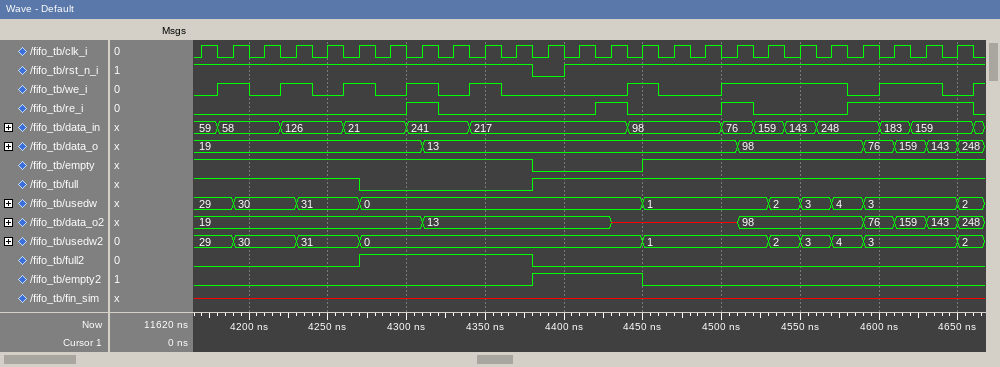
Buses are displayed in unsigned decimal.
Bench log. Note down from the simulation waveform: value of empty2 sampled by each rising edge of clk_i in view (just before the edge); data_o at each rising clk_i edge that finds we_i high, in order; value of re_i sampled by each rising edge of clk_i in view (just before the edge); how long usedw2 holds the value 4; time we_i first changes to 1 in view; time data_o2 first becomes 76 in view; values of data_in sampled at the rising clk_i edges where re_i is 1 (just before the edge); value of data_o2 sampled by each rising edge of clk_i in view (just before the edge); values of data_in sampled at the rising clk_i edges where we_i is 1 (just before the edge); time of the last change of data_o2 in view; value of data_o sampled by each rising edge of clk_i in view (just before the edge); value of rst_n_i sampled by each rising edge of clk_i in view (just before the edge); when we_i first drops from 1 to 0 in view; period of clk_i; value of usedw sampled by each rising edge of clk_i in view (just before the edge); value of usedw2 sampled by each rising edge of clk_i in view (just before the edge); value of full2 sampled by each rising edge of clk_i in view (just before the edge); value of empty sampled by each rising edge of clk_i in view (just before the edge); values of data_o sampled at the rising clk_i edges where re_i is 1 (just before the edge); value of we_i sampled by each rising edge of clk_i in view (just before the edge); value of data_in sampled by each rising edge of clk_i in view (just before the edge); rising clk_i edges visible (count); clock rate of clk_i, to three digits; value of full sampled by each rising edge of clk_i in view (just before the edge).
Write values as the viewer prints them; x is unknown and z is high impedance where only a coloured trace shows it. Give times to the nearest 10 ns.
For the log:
0 0 0 0 0 0 0 0 0 0 0 1 1 1 1 0 0 0 0 0 0 0 0 0 0
19, 19, 19, 19, 13, 13, 13, 98, 98, 98, 76, 159
0 0 0 0 0 0 0 1 0 0 0 0 0 1 0 0 0 1 0 0 0 1 1 1 1
20 ns
4180 ns
4590 ns
241, 217, 76, 248, 183, 159, 159
19, 19, 19, 19, 19, 19, 19, 19, 13, 13, 13, 13, 13, 13, x, x, x, x, 98, 98, 98, 98, 76, 159, 143
58, 126, 21, 241, 217, 98, 76, 159, 143, 248, 183, 159
4650 ns
19, 19, 19, 19, 19, 19, 19, 19, 13, 13, 13, 13, 13, 13, 13, 13, 13, 13, 98, 98, 98, 98, 76, 159, 143
1 1 1 1 1 1 1 1 1 1 1 0 1 1 1 1 1 1 1 1 1 1 1 1 1
4200 ns
20 ns
29, 29, 30, 30, 31, 31, 0, 0, 0, 0, 0, 0, 0, 0, 0, 1, 1, 1, 1, 2, 3, 4, 3, 3, 3
29, 29, 30, 30, 31, 31, 0, 0, 0, 0, 0, 0, 0, 0, 0, 1, 1, 1, 1, 2, 3, 4, 3, 3, 3
0 0 0 0 0 0 1 1 1 1 1 0 0 0 0 0 0 0 0 0 0 0 0 0 0
1 1 1 1 1 1 1 1 1 1 1 0 0 0 0 1 1 1 1 1 1 1 1 1 1
19, 13, 13, 98, 76, 159, 143
0 1 0 1 0 1 0 1 0 1 0 0 0 0 1 0 0 1 1 1 1 0 1 1 0
59, 58, 58, 126, 126, 21, 21, 241, 241, 217, 217, 217, 217, 217, 98, 98, 98, 76, 159, 143, 248, 248, 183, 159, 159
25
50.0 MHz
1 1 1 1 1 1 0 0 0 0 0 1 1 1 1 1 1 1 1 1 1 1 1 1 1
